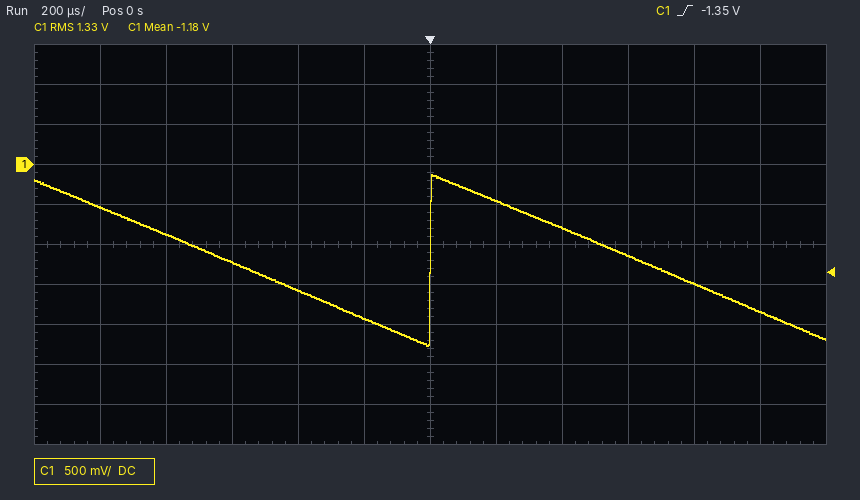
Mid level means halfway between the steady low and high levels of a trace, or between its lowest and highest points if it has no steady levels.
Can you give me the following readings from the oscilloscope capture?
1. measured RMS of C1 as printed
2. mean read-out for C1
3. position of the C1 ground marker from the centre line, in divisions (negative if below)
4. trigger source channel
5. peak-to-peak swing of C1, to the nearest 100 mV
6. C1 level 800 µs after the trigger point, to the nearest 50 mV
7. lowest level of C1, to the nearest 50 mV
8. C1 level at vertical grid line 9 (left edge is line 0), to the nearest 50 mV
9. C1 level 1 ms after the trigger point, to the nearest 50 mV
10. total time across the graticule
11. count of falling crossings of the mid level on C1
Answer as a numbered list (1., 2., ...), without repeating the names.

1. 1.33 V
2. -1.18 V
3. +2.0 div
4. C1
5. 2.10 V
6. -1.50 V
7. -2.25 V
8. -1.15 V
9. -1.85 V
10. 2.4 ms
11. 2
